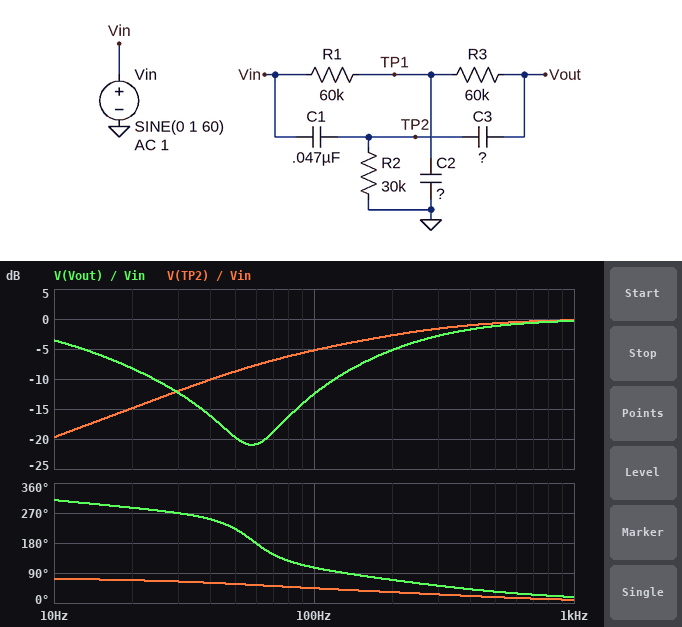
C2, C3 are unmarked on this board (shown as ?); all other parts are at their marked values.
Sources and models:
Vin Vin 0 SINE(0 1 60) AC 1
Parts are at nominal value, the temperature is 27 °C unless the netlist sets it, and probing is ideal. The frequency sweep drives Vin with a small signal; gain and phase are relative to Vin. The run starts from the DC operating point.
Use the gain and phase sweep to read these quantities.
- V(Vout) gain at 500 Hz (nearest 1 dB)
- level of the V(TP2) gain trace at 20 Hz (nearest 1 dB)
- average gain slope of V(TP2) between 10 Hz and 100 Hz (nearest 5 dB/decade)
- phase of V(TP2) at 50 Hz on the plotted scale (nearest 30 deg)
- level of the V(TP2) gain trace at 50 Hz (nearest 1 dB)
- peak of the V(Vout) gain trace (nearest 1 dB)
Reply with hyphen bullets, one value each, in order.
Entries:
- -1 dB
- -15 dB
- 15 dB/decade
- 60 deg
- -9 dB
- 0 dB
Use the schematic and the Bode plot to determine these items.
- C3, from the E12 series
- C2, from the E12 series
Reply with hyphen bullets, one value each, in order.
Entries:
- 18 nF
- 270 nF
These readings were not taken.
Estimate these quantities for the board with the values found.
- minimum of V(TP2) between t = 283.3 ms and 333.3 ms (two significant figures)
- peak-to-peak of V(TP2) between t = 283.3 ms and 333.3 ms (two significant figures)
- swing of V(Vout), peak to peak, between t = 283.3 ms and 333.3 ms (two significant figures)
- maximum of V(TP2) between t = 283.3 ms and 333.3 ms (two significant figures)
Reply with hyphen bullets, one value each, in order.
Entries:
- -410 mV
- 830 mV
- 180 mV
- 410 mV
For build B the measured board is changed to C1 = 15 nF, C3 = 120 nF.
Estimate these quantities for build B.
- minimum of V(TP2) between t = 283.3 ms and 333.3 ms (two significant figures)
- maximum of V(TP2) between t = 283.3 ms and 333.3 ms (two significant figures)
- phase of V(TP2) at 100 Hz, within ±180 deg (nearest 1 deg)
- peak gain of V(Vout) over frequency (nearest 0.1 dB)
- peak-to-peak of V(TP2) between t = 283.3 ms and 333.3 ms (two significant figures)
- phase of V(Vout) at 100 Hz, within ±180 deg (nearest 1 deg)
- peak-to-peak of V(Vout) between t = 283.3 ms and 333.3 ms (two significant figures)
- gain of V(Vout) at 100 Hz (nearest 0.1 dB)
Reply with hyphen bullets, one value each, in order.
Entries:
- -84 mV
- 84 mV
- 69 deg
- 0 dB
- 170 mV
- 88 deg
- 93 mV
- -16.9 dB
